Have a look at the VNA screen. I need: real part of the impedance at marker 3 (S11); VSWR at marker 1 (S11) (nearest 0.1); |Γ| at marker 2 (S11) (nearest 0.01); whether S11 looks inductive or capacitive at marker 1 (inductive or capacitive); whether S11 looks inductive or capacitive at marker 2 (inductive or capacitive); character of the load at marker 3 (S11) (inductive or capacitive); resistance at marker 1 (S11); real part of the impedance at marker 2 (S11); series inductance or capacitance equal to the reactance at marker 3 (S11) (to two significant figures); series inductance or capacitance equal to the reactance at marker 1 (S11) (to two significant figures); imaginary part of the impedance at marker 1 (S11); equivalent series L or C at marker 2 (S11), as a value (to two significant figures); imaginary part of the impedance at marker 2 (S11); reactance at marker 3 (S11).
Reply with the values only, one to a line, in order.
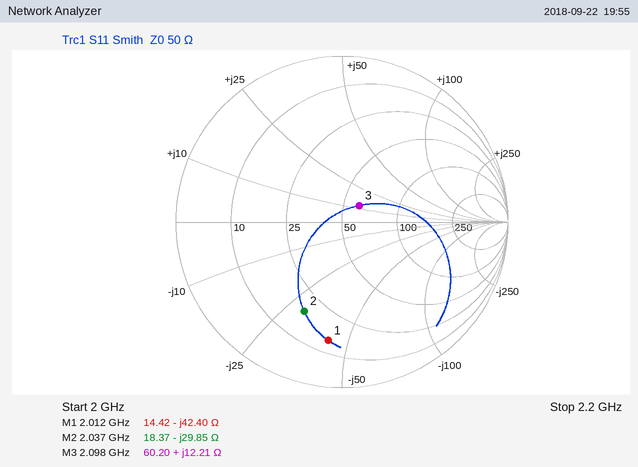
60.20 Ω
6.1
0.58
capacitive
capacitive
inductive
14.42 Ω
18.37 Ω
930 pH
1.9 pF
-42.40 Ω
2.6 pF
-29.85 Ω
+12.21 Ω
